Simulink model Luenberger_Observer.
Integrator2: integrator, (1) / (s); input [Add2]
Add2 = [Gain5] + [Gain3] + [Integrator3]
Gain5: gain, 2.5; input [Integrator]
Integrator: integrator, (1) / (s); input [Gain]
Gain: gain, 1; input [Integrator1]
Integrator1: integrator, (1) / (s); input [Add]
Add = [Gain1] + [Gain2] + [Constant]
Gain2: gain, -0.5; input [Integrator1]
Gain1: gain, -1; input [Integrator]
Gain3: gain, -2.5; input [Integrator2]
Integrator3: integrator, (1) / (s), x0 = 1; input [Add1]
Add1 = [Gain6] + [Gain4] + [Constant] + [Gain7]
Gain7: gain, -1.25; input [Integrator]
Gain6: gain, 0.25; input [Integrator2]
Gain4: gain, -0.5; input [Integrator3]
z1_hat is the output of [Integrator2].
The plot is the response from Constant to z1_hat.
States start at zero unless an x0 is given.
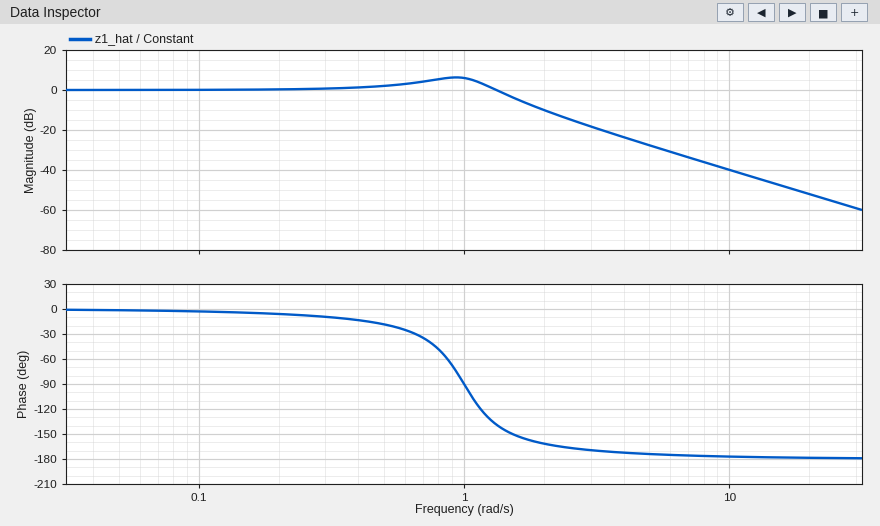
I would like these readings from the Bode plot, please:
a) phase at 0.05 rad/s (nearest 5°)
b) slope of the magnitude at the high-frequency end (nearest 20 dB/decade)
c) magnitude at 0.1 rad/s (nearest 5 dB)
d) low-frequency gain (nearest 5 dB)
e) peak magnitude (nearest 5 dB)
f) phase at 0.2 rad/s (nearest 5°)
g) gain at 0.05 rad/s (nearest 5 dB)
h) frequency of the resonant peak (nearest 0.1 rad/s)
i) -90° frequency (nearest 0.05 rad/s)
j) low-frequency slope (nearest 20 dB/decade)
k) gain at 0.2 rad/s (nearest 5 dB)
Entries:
0°
-40 dB/decade
0 dB
0 dB
5 dB
-5°
0 dB
0.9 rad/s
1.00 rad/s
0 dB/decade
0 dB
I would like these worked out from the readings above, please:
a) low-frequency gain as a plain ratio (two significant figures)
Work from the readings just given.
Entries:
1.0
